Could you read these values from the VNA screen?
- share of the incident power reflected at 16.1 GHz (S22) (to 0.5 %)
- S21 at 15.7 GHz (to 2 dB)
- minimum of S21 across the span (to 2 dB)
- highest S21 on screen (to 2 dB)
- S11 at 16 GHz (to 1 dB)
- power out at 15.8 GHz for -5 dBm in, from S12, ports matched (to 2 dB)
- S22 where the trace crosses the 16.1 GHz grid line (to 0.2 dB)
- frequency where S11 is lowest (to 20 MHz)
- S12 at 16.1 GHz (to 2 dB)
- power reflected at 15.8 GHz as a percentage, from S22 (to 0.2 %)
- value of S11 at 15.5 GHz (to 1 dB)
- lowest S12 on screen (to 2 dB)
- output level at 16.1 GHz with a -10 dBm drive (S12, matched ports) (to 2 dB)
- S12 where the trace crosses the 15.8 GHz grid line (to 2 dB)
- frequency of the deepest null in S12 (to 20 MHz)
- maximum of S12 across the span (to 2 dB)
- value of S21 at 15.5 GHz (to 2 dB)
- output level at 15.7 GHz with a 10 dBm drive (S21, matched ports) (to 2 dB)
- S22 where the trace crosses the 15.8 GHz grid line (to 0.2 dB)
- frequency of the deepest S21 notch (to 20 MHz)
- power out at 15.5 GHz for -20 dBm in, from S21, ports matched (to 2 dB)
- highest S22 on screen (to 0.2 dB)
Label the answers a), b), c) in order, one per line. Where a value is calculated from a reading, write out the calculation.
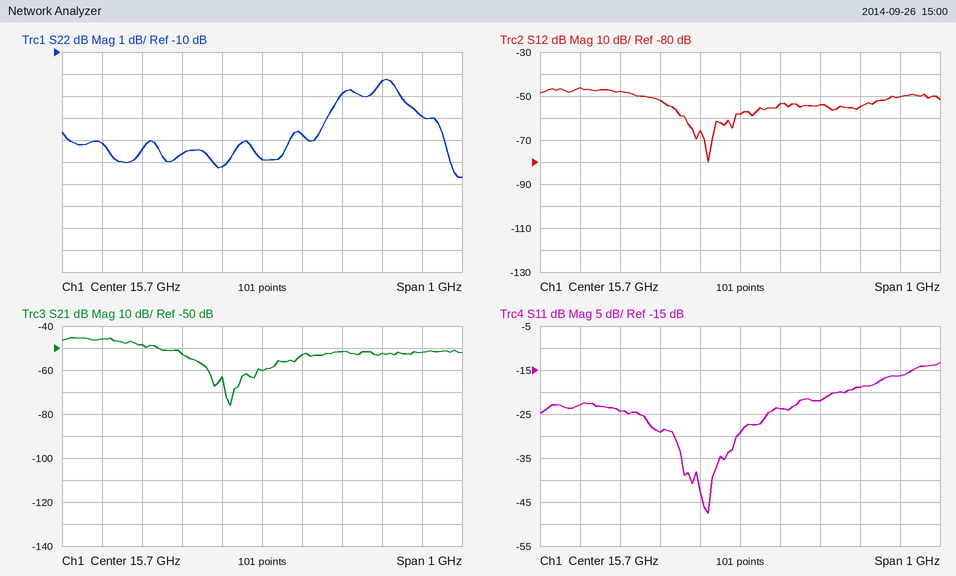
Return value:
a) 10^(-13/10) ≈ 5.0 %
b) -60 dB
c) -76 dB
d) -46 dB
e) -19 dB
f) -5 dBm + (-54 dB) = -58 dBm
g) -13.0 dB
h) 15.62 GHz
i) -50 dB
j) 10^(-13.8/10) ≈ 4.2 %
k) -29 dB
l) -80 dB
m) -10 dBm + (-50 dB) = -60 dBm
n) -54 dB
o) 15.62 GHz
p) -46 dB
q) -52 dB
r) 10 dBm + (-60 dB) = -50 dBm
s) -13.8 dB
t) 15.62 GHz
u) -20 dBm + (-52 dB) = -72 dBm
v) -11.2 dB
